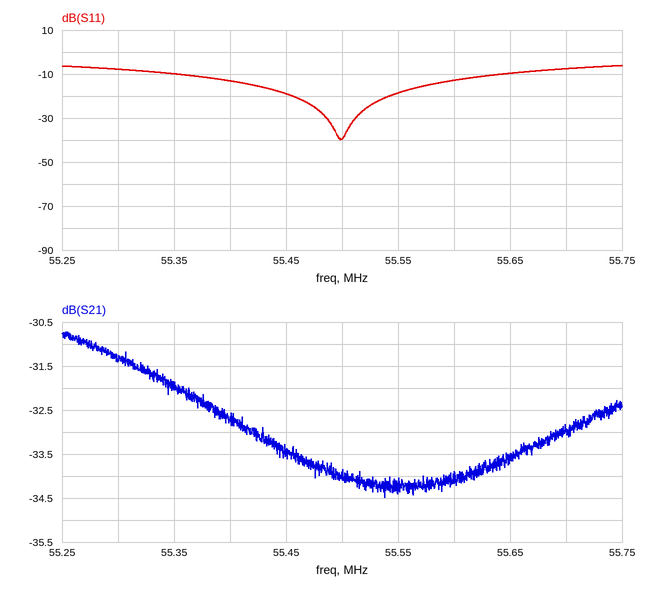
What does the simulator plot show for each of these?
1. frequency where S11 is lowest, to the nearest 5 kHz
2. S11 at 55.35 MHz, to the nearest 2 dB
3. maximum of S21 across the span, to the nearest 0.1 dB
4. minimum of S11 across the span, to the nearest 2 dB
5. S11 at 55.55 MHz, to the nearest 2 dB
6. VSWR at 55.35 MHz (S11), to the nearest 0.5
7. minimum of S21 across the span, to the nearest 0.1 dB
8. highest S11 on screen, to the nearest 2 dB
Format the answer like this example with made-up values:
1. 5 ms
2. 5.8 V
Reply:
1. 55.500 MHz
2. -10 dB
3. -30.7 dB
4. -40 dB
5. -18 dB
6. 2.0
7. -34.5 dB
8. -6 dB
